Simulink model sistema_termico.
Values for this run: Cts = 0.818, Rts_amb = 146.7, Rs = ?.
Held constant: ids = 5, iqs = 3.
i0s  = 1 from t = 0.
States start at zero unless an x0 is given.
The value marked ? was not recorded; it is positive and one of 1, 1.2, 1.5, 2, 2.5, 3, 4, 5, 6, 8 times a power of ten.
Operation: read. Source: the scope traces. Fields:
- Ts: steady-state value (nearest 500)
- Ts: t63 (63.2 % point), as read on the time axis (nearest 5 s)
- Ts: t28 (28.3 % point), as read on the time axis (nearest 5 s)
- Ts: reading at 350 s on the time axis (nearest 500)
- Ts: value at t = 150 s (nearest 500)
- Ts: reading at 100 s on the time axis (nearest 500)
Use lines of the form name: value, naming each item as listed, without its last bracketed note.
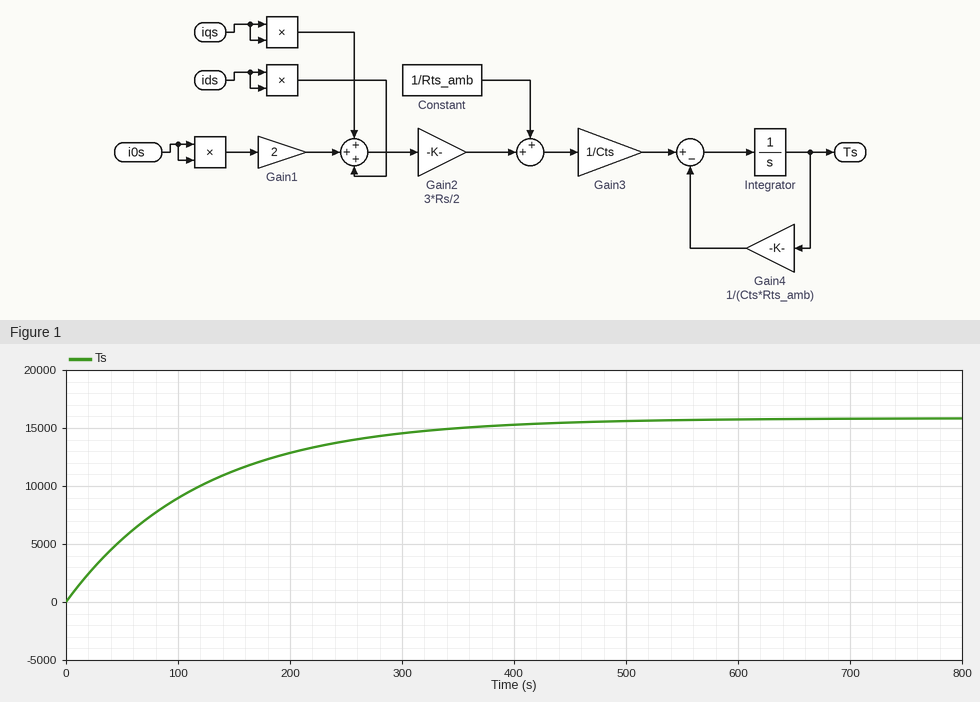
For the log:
Ts: steady-state value: 16000
Ts: t63 (63.2 % point), as read on the time axis: 120 s
Ts: t28 (28.3 % point), as read on the time axis: 40 s
Ts: reading at 350 s on the time axis: 15000
Ts: value at t = 150 s: 11500
Ts: reading at 100 s on the time axis: 9000
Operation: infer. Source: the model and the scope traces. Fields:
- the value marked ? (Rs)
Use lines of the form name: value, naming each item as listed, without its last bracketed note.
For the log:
the value marked ?: 2
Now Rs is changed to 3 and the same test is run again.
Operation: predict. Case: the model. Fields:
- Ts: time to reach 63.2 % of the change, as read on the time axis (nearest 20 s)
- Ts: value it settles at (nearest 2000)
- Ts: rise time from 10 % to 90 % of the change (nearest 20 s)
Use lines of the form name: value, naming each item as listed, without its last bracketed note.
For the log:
Ts: time to reach 63.2 % of the change, as read on the time axis: 120 s
Ts: value it settles at: 24000
Ts: rise time from 10 % to 90 % of the change: 260 s
